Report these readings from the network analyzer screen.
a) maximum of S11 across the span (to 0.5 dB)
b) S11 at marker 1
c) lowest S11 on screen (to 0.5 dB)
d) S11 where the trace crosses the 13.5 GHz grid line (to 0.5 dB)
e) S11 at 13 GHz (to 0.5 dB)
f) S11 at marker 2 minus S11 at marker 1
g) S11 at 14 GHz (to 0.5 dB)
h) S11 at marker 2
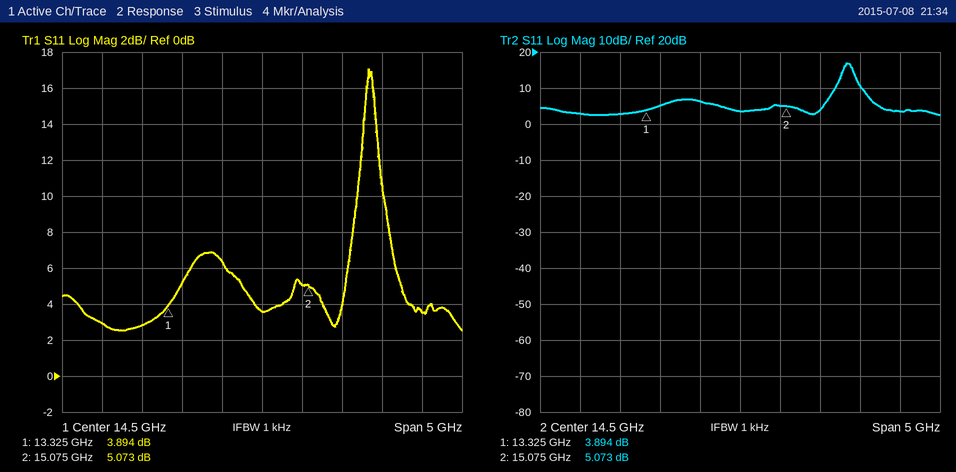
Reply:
17.0 dB
3.894 dB
2.5 dB
5.0 dB
3.0 dB
1.179 dB
6.5 dB
5.073 dB
